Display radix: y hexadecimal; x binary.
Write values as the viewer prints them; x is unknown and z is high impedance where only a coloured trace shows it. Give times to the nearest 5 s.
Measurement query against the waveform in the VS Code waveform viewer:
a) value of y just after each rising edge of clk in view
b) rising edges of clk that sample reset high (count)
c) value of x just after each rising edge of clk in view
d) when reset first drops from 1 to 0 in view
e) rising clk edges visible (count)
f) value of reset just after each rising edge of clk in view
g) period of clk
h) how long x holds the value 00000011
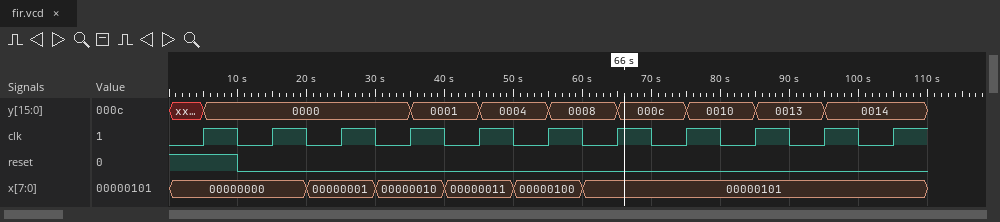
0000, 0000, 0000, 0001, 0004, 0008, 000c, 0010, 0013, 0014, 0014
1
00000000, 00000000, 00000001, 00000010, 00000011, 00000100, 00000101, 00000101, 00000101, 00000101, 00000101
10 s
11
1 0 0 0 0 0 0 0 0 0 0
10 s
10 s
